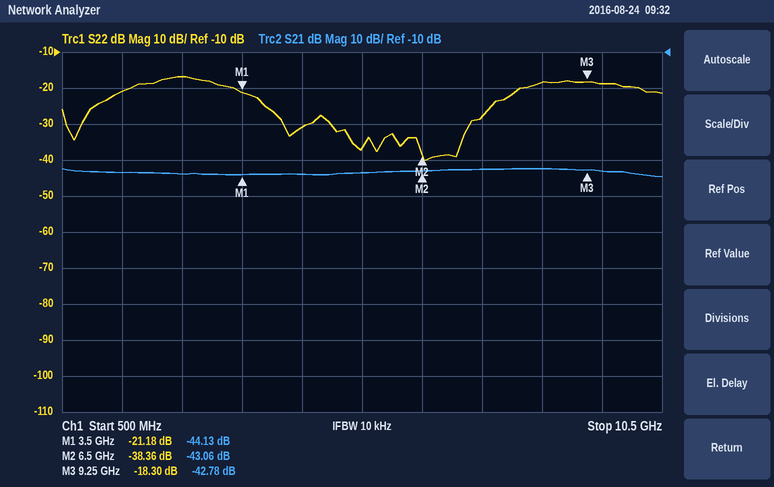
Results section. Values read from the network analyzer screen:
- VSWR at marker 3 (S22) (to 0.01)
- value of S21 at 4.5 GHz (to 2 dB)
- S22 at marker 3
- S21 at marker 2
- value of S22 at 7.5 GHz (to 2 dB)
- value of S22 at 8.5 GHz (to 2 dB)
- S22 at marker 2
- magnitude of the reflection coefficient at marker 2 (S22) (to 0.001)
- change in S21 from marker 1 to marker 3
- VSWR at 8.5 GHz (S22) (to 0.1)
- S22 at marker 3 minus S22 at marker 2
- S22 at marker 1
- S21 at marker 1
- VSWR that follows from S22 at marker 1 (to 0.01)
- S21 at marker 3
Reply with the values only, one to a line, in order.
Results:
1.28
-44 dB
-18.30 dB
-43.06 dB
-28 dB
-18 dB
-38.36 dB
0.012
1.35 dB
1.3
20.06 dB
-21.18 dB
-44.13 dB
1.19
-42.78 dB
